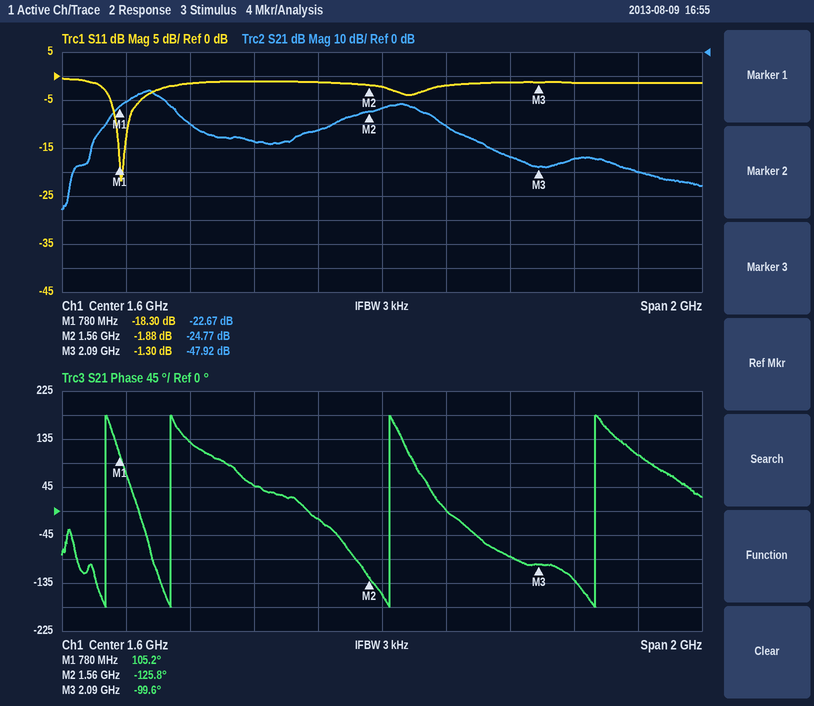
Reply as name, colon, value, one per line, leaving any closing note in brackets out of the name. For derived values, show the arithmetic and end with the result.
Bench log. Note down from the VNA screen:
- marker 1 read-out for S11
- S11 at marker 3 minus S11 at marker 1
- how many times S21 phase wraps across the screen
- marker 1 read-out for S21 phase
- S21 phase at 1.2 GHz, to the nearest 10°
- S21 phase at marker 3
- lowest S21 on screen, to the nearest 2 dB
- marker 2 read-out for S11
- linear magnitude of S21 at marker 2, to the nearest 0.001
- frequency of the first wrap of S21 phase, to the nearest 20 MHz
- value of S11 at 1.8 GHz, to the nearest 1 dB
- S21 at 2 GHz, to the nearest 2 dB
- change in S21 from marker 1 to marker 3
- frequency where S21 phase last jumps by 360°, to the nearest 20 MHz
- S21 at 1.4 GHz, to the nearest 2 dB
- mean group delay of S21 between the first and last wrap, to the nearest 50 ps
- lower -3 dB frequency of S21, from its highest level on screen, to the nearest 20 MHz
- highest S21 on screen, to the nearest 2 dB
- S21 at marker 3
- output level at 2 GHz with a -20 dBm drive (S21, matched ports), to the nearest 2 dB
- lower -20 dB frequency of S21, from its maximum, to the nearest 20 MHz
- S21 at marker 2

marker 1 read-out for S11: -18.30 dB
S11 at marker 3 minus S11 at marker 1: -1.3 − (-18.3) = 17.00 dB
how many times S21 phase wraps across the screen: 4
marker 1 read-out for S21 phase: 105.2°
S21 phase at 1.2 GHz, to the nearest 10°: 50°
S21 phase at marker 3: -99.6°
lowest S21 on screen, to the nearest 2 dB: -66 dB
marker 2 read-out for S11: -1.88 dB
linear magnitude of S21 at marker 2, to the nearest 0.001: 10^(-24.77/20) ≈ 0.058
frequency of the first wrap of S21 phase, to the nearest 20 MHz: 740 MHz
value of S11 at 1.8 GHz, to the nearest 1 dB: -2 dB
S21 at 2 GHz, to the nearest 2 dB: -44 dB
change in S21 from marker 1 to marker 3: -47.92 − (-22.67) = -25.25 dB
frequency where S21 phase last jumps by 360°, to the nearest 20 MHz: 2.26 GHz
S21 at 1.4 GHz, to the nearest 2 dB: -32 dB
mean group delay of S21 between the first and last wrap, to the nearest 50 ps: 3 cycles / (2.26 GHz − 740 MHz) ≈ 1.97 ns, so 1.95 ns to the nearest 50 ps
lower -3 dB frequency of S21, from its highest level on screen, to the nearest 20 MHz: 820 MHz
highest S21 on screen, to the nearest 2 dB: -16 dB
S21 at marker 3: -47.92 dB
output level at 2 GHz with a -20 dBm drive (S21, matched ports), to the nearest 2 dB: -20 dBm + (-44 dB) = -64 dBm
lower -20 dB frequency of S21, from its maximum, to the nearest 20 MHz: 700 MHz
S21 at marker 2: -24.77 dB
